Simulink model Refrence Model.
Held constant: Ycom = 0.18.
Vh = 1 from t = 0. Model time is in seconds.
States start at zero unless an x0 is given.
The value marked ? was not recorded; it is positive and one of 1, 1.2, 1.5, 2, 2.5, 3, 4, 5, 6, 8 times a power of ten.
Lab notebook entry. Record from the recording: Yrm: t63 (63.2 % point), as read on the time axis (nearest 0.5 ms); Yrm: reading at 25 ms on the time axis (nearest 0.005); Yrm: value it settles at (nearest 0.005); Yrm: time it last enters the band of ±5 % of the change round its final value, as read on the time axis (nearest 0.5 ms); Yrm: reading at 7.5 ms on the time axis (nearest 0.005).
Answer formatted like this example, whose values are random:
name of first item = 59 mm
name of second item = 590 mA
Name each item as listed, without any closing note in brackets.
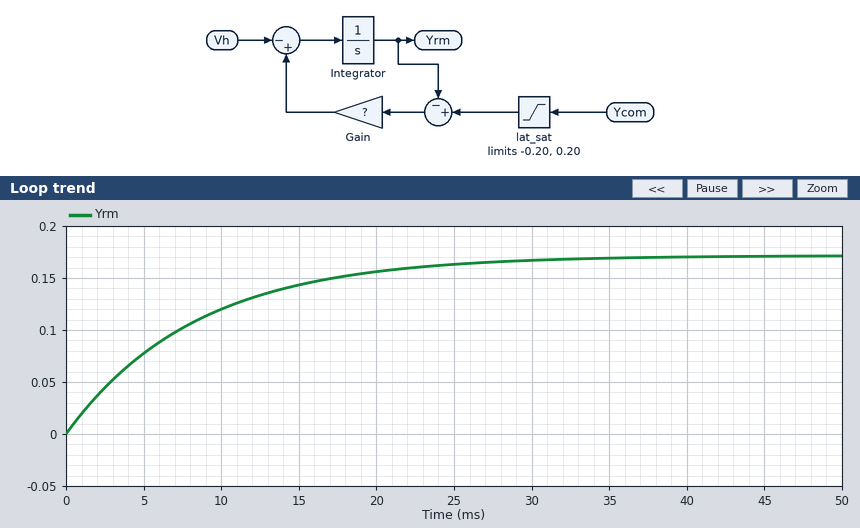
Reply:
Yrm: t63 (63.2 % point), as read on the time axis = 8.5 ms
Yrm: reading at 25 ms on the time axis = 0.165
Yrm: value it settles at = 0.170
Yrm: time it last enters the band of ±5 % of the change round its final value, as read on the time axis = 25.0 ms
Yrm: reading at 7.5 ms on the time axis = 0.100
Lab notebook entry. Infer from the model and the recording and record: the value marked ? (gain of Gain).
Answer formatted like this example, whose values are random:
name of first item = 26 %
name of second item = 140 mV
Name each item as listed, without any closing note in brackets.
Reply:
the value marked ? = 120
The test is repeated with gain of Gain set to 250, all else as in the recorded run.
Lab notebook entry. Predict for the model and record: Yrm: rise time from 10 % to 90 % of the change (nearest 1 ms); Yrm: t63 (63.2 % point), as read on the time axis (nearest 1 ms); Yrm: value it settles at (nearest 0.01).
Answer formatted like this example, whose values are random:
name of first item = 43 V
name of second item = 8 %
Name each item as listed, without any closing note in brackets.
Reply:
Yrm: rise time from 10 % to 90 % of the change = 9 ms
Yrm: t63 (63.2 % point), as read on the time axis = 4 ms
Yrm: value it settles at = 0.18
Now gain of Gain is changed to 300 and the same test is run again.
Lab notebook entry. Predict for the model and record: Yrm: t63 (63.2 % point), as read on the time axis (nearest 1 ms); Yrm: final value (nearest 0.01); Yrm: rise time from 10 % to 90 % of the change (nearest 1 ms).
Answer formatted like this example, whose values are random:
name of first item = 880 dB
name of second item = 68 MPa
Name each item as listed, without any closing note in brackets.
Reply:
Yrm: t63 (63.2 % point), as read on the time axis = 3 ms
Yrm: final value = 0.18
Yrm: rise time from 10 % to 90 % of the change = 7 ms
